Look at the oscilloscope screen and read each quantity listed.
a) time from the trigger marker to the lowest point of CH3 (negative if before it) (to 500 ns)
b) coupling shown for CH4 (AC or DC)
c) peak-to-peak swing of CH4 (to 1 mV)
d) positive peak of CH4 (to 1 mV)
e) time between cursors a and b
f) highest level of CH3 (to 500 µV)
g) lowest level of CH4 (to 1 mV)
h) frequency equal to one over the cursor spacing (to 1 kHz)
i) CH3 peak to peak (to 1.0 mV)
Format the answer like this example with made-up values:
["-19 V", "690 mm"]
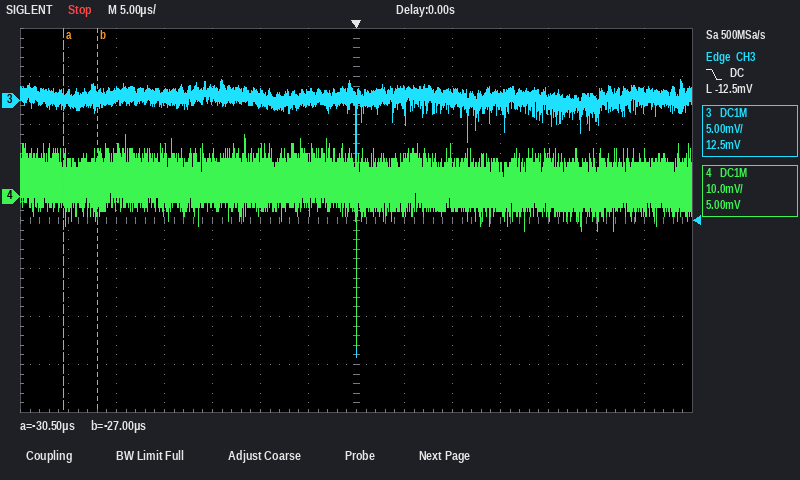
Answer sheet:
["0.0 µs", "DC", "44 mV", "13 mV", "3.5 µs", "2.0 mV", "-31 mV", "286 kHz", "29.0 mV"]
